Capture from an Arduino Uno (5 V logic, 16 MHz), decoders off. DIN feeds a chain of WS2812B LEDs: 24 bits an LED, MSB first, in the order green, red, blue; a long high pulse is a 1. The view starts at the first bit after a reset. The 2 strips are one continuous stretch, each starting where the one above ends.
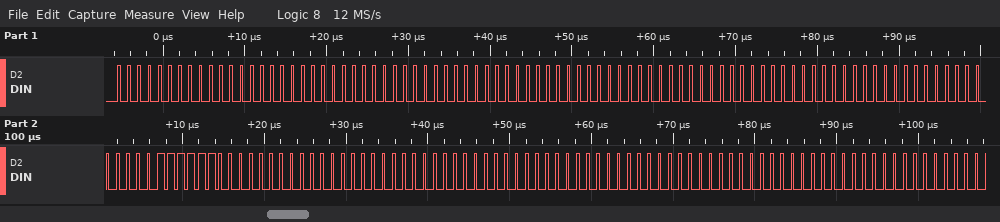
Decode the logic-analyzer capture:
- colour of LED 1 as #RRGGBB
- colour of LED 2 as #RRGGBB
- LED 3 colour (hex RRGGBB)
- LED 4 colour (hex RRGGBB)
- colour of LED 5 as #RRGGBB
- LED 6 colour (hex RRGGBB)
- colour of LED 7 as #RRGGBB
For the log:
#000000
#000000
#000000
#00003F
#000000
#000000
#000000
